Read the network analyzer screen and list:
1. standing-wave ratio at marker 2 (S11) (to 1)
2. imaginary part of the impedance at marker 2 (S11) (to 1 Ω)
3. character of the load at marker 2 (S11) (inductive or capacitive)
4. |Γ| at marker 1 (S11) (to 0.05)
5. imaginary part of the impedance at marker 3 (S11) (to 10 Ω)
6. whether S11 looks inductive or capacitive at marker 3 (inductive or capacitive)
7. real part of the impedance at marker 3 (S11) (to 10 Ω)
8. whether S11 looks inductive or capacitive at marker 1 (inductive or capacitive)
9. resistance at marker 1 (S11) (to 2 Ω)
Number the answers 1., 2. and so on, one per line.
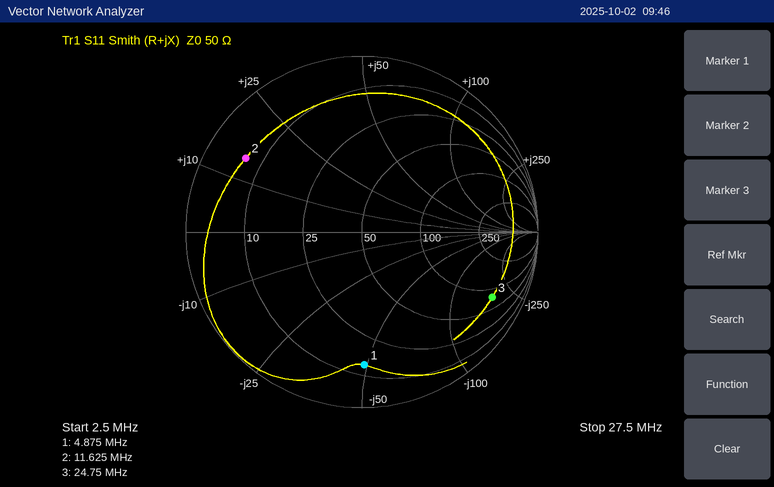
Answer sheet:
1. 8
2. +14 Ω
3. inductive
4. 0.75
5. -180 Ω
6. capacitive
7. 80 Ω
8. capacitive
9. 14 Ω
